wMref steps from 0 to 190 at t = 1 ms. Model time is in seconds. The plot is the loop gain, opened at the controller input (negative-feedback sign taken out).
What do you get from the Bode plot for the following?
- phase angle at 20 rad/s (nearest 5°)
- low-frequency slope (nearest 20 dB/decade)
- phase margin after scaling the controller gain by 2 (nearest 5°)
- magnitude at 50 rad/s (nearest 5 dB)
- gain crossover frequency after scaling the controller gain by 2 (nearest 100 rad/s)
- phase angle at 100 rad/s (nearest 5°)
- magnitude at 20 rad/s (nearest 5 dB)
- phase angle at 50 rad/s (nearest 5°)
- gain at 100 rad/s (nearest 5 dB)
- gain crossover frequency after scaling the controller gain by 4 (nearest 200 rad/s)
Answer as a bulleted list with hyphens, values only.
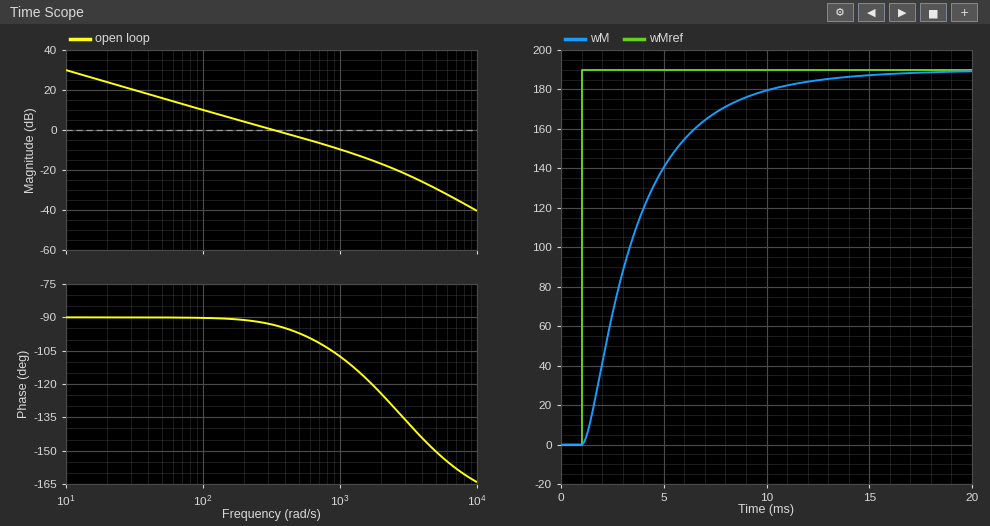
- -90°
- -20 dB/decade
- 80°
- 15 dB
- 700 rad/s
- -90°
- 25 dB
- -90°
- 10 dB
- 1200 rad/s
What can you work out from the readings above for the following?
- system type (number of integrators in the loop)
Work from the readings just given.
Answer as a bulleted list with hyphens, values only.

- 1
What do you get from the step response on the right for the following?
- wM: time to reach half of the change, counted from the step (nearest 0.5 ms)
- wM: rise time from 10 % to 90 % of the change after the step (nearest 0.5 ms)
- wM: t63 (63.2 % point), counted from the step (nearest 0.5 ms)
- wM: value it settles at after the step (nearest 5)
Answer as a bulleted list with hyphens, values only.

- 2.0 ms
- 6.5 ms
- 3.0 ms
- 190
